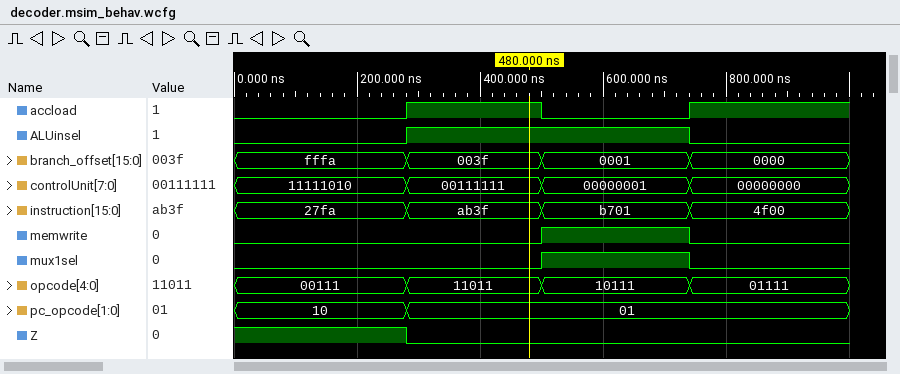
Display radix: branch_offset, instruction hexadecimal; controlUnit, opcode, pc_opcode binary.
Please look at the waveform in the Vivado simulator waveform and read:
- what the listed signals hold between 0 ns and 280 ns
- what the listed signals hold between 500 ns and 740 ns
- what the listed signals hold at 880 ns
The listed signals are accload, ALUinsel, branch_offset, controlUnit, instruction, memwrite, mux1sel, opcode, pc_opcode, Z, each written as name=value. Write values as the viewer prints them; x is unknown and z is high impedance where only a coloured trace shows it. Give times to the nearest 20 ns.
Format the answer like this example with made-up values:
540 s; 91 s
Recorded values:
accload=0, ALUinsel=0, branch_offset=fffa, controlUnit=11111010, instruction=27fa, memwrite=0, mux1sel=0, opcode=00111, pc_opcode=10, Z=1; accload=0, ALUinsel=1, branch_offset=0001, controlUnit=00000001, instruction=b701, memwrite=1, mux1sel=1, opcode=10111, pc_opcode=01, Z=0; accload=1, ALUinsel=0, branch_offset=0000, controlUnit=00000000, instruction=4f00, memwrite=0, mux1sel=0, opcode=01111, pc_opcode=01, Z=0
